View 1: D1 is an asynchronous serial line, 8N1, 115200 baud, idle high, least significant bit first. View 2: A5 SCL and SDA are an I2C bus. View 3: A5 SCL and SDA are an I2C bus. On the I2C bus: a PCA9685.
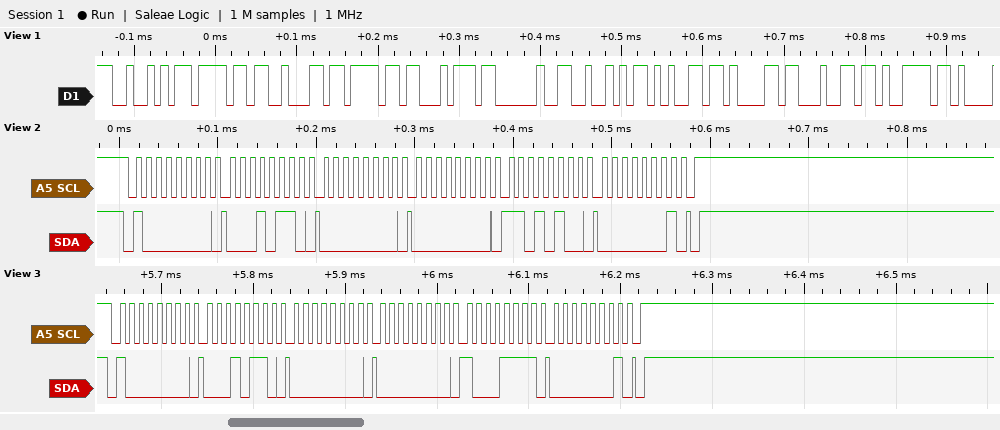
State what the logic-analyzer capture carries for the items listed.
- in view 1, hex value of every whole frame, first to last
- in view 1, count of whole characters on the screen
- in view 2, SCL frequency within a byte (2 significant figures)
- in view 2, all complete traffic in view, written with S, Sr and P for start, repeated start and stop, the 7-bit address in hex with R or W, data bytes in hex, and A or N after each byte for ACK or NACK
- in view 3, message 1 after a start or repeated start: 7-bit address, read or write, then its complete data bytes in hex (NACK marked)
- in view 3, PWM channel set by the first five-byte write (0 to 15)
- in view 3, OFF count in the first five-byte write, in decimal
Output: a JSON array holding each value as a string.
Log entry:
["52 6F 62 6F 74 20 52 65 61 64 79", "11", "100 kHz", "S 40W A 16 A 00 A 00 A D4 A 01 A P", "0x40 write: 16 00 00 8F 01", "4", "399"]
